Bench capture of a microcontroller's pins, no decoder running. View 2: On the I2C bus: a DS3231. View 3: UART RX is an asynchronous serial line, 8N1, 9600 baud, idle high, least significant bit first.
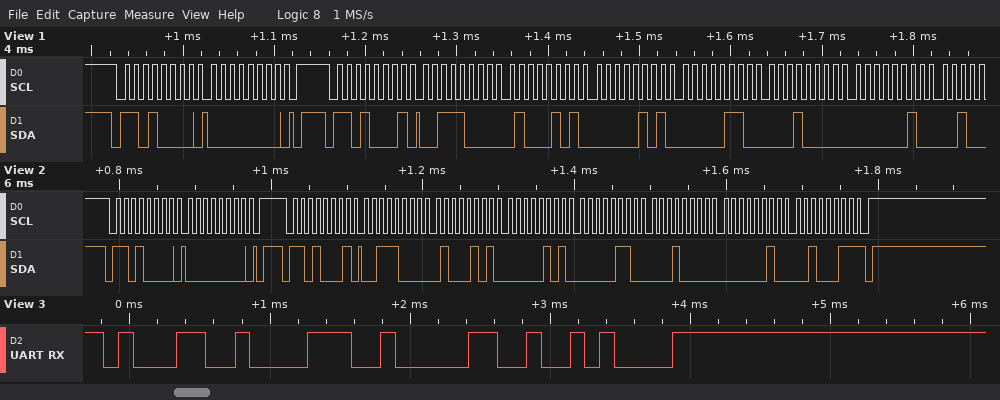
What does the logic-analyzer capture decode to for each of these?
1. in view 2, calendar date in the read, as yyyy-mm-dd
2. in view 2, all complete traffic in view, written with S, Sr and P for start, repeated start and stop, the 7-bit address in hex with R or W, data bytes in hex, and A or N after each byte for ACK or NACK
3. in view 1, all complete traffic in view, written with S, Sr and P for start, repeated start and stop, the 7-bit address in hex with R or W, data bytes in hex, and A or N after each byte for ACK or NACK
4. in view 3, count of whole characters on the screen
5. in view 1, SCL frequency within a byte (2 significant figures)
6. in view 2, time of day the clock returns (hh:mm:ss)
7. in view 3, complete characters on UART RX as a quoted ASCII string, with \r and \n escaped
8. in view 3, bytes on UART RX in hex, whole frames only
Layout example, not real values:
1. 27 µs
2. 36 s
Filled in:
1. 2023-02-10
2. S 68W A 00 A P S 68R A 38 A 45 A 05 A 06 A 10 A 02 A 23 N P
3. S 68W A 00 A P S 68R A 38 A 45 A 05 A 06 A 10 A 02 A
4. 4
5. 100 kHz
6. 05:45:38
7. "180\n"
8. 0x31 0x38 0x30 0x0A
